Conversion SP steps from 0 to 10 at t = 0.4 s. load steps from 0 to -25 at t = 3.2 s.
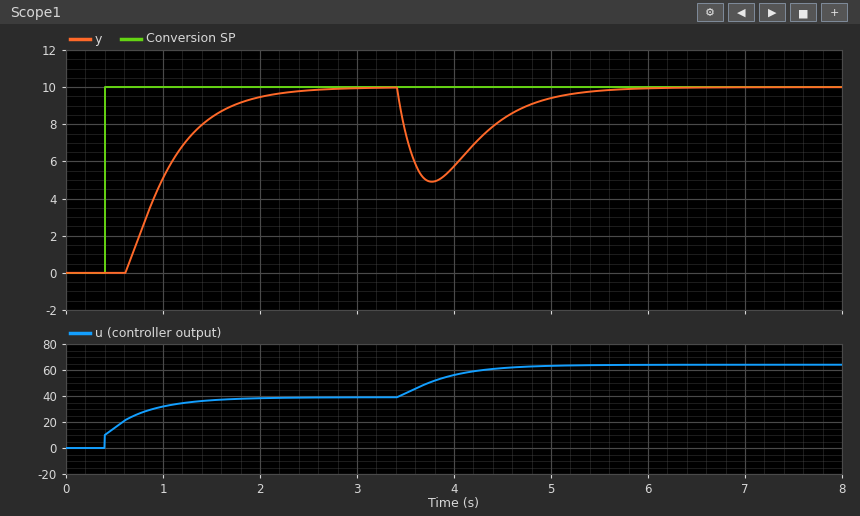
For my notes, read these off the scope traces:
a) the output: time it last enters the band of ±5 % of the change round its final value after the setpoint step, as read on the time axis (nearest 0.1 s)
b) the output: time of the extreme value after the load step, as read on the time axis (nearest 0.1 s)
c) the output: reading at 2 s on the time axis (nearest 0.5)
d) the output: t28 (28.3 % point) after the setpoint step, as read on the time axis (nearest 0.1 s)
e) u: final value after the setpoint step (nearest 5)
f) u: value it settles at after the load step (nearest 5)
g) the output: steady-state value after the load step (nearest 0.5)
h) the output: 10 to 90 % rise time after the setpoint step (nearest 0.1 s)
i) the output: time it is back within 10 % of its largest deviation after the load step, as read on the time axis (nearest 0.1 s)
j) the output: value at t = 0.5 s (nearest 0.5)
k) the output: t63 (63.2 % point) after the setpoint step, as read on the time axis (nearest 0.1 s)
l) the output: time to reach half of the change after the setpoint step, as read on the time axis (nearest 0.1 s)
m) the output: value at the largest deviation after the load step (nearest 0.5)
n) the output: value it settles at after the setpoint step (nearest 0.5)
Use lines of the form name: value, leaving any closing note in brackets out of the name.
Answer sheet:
the output: time it last enters the band of ±5 % of the change round its final value after the setpoint step, as read on the time axis: 2.0 s
the output: time of the extreme value after the load step, as read on the time axis: 3.8 s
the output: reading at 2 s on the time axis: 9.5
the output: t28 (28.3 % point) after the setpoint step, as read on the time axis: 0.8 s
u: final value after the setpoint step: 40
u: value it settles at after the load step: 65
the output: steady-state value after the load step: 10.0
the output: 10 to 90 % rise time after the setpoint step: 1.0 s
the output: time it is back within 10 % of its largest deviation after the load step, as read on the time axis: 5.1 s
the output: value at t = 0.5 s: 0.0
the output: t63 (63.2 % point) after the setpoint step, as read on the time axis: 1.1 s
the output: time to reach half of the change after the setpoint step, as read on the time axis: 1.0 s
the output: value at the largest deviation after the load step: 5.0
the output: value it settles at after the setpoint step: 10.0
